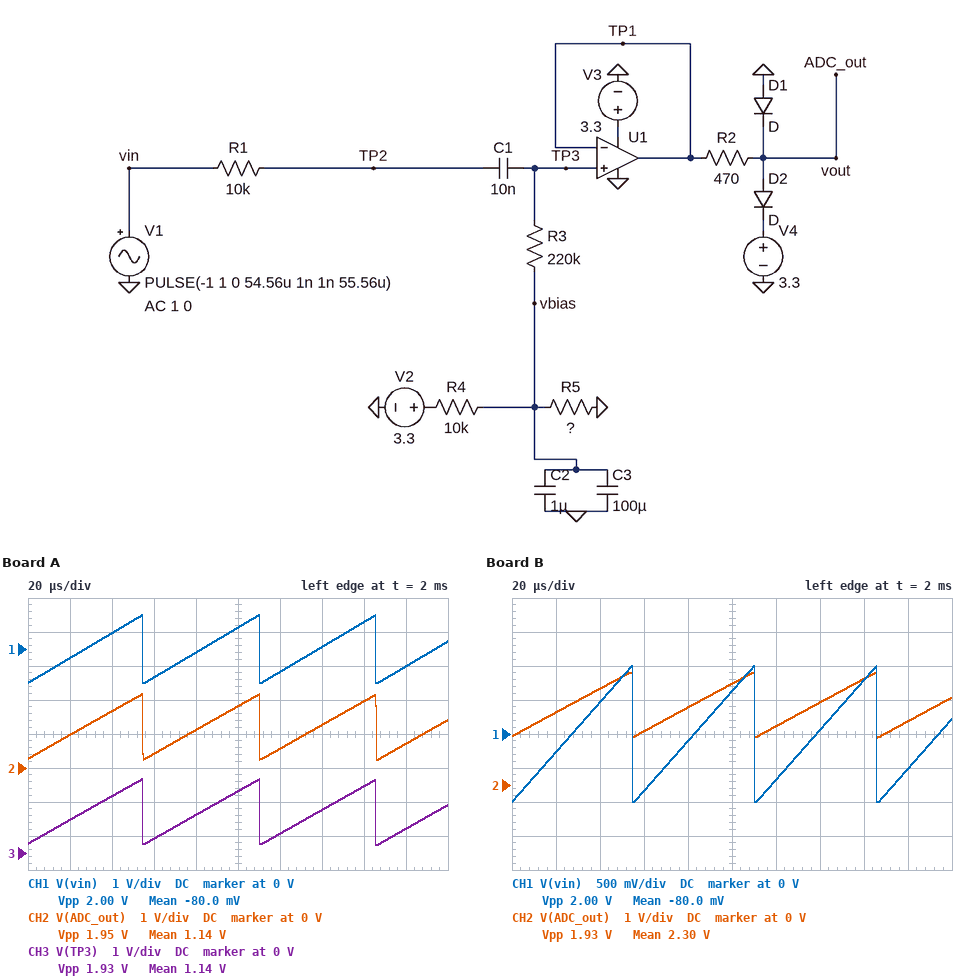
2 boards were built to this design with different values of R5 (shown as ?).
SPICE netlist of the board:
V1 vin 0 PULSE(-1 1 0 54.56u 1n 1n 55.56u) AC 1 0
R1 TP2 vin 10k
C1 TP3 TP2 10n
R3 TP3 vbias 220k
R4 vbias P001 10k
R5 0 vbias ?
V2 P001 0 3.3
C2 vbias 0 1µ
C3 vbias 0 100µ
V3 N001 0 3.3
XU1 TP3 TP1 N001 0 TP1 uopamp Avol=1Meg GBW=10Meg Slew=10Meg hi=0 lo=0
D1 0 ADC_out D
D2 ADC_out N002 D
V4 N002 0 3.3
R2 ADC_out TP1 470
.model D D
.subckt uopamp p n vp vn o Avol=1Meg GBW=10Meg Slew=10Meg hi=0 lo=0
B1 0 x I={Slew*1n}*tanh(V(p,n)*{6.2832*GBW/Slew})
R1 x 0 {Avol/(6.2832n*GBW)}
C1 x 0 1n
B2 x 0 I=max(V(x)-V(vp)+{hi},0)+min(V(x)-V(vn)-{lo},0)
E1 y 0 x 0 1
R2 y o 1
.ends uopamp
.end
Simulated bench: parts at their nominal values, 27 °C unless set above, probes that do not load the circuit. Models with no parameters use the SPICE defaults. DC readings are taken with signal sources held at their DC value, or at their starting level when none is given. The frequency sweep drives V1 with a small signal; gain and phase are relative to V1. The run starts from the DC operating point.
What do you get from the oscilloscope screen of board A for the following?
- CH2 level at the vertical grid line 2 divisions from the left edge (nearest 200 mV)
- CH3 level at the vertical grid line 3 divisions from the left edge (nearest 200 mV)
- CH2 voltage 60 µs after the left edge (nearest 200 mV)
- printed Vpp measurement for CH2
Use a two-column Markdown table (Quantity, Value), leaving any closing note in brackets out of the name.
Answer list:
| Quantity | Value |
|---|---|
| CH2 level at the vertical grid line 2 divisions from the left edge | 1.6 V |
| CH3 level at the vertical grid line 3 divisions from the left edge | 400 mV |
| CH2 voltage 60 µs after the left edge | 400 mV |
| printed Vpp measurement for CH2 | 1.95 V |
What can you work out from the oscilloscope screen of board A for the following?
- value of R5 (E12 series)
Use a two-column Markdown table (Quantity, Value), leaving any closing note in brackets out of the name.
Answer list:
| Quantity | Value |
|---|---|
| value of R5 | 3.3 kΩ |
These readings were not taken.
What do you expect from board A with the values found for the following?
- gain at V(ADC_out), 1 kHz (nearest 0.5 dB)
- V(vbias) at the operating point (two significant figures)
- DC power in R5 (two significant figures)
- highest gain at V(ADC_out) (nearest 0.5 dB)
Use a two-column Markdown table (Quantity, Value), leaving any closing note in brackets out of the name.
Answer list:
| Quantity | Value |
|---|---|
| gain at V(ADC_out), 1 kHz | -0.5 dB |
| V(vbias) at the operating point | 820 mV |
| DC power in R5 | 200 µW |
| highest gain at V(ADC_out) | -0.5 dB |
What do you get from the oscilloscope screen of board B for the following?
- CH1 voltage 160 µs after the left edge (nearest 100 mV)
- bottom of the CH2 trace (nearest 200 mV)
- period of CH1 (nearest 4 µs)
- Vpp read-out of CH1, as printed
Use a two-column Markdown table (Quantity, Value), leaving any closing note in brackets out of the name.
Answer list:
| Quantity | Value |
|---|---|
| CH1 voltage 160 µs after the left edge | 800 mV |
| bottom of the CH2 trace | 1.4 V |
| period of CH1 | 56 µs |
| Vpp read-out of CH1, as printed | 2.00 V |
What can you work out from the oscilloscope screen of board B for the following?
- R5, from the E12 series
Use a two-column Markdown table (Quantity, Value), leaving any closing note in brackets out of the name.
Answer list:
| Quantity | Value |
|---|---|
| R5, from the E12 series | 15 kΩ |
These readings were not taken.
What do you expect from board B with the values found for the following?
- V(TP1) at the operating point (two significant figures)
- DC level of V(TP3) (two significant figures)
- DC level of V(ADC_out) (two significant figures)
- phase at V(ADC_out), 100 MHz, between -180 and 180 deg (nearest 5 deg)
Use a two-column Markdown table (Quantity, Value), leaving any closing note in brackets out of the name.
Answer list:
| Quantity | Value |
|---|---|
| V(TP1) at the operating point | 2.0 V |
| DC level of V(TP3) | 2.0 V |
| DC level of V(ADC_out) | 2.0 V |
| phase at V(ADC_out), 100 MHz, between -180 and 180 deg | -85 deg |
